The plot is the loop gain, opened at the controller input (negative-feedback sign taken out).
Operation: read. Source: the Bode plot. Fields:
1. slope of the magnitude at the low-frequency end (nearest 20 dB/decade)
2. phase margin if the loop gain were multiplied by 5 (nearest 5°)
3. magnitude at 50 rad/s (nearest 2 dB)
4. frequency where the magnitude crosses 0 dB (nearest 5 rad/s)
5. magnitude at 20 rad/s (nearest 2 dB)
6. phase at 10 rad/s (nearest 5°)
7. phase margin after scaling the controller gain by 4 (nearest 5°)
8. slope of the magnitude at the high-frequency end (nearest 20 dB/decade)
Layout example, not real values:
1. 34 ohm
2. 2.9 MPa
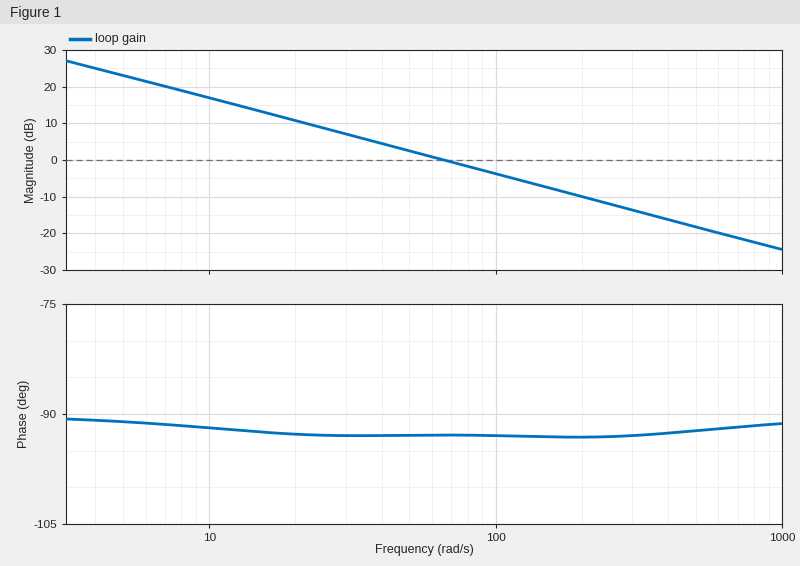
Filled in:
1. -20 dB/decade
2. 85°
3. 2 dB
4. 65 rad/s
5. 10 dB
6. -90°
7. 85°
8. -20 dB/decade
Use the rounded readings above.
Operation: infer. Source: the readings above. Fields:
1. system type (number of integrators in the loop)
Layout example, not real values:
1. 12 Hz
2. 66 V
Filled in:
1. 1
